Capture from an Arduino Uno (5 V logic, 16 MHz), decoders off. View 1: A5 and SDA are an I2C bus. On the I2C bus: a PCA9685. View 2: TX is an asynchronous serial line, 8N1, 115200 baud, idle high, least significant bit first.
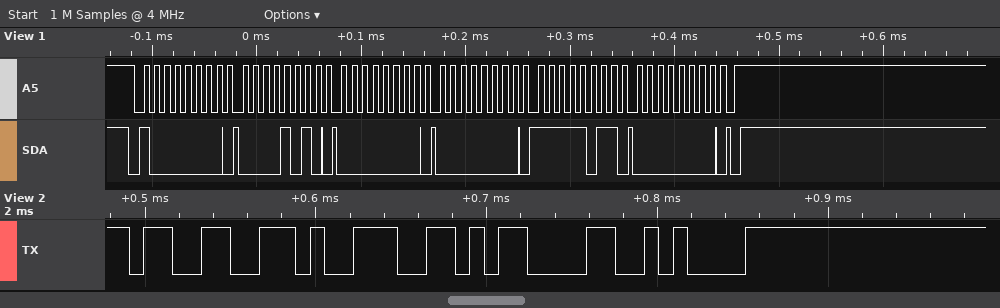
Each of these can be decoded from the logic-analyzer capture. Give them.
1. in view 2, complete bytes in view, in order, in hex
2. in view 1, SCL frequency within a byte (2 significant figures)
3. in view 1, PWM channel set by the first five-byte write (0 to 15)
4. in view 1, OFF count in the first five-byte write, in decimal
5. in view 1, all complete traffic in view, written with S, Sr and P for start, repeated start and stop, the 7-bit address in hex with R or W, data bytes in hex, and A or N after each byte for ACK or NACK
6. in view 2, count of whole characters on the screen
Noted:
0x33 0x39 0x0D 0x0A
100 kHz
1
251
S 40W A 0A A 00 A 00 A FB A 00 A P
4
